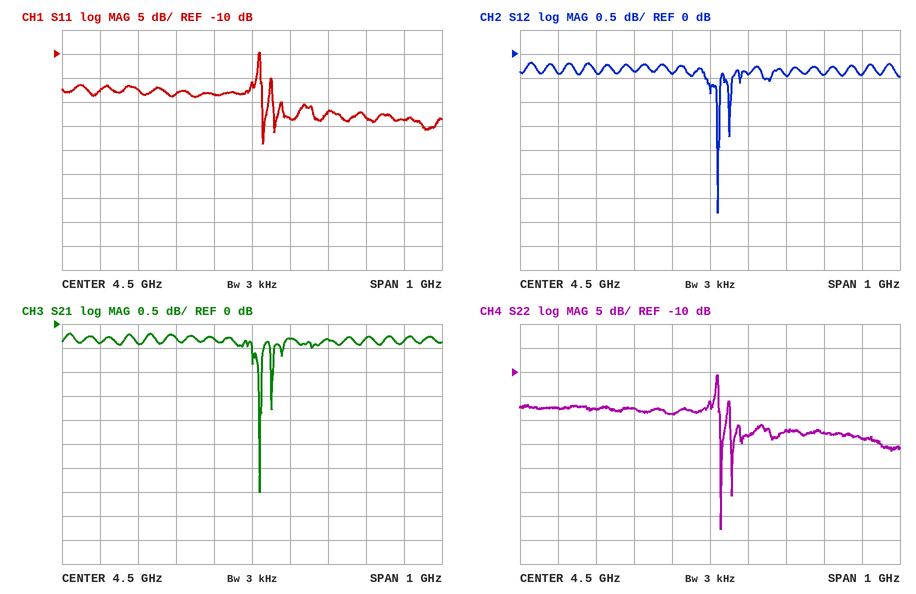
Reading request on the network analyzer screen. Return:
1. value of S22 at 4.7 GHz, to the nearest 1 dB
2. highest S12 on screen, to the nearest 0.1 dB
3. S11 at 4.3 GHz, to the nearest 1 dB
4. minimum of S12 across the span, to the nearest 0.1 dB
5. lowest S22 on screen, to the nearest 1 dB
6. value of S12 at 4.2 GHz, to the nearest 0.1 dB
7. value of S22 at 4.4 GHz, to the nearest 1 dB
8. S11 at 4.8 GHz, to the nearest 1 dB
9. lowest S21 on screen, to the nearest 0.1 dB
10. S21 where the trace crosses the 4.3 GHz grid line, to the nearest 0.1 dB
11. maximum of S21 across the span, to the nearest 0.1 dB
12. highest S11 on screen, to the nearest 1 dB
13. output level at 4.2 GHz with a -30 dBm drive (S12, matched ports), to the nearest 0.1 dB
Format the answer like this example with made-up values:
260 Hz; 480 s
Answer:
-22 dB; -0.2 dB; -18 dB; -3.3 dB; -43 dB; -0.4 dB; -19 dB; -23 dB; -3.5 dB; -0.3 dB; -0.2 dB; -10 dB; -30.4 dBm
